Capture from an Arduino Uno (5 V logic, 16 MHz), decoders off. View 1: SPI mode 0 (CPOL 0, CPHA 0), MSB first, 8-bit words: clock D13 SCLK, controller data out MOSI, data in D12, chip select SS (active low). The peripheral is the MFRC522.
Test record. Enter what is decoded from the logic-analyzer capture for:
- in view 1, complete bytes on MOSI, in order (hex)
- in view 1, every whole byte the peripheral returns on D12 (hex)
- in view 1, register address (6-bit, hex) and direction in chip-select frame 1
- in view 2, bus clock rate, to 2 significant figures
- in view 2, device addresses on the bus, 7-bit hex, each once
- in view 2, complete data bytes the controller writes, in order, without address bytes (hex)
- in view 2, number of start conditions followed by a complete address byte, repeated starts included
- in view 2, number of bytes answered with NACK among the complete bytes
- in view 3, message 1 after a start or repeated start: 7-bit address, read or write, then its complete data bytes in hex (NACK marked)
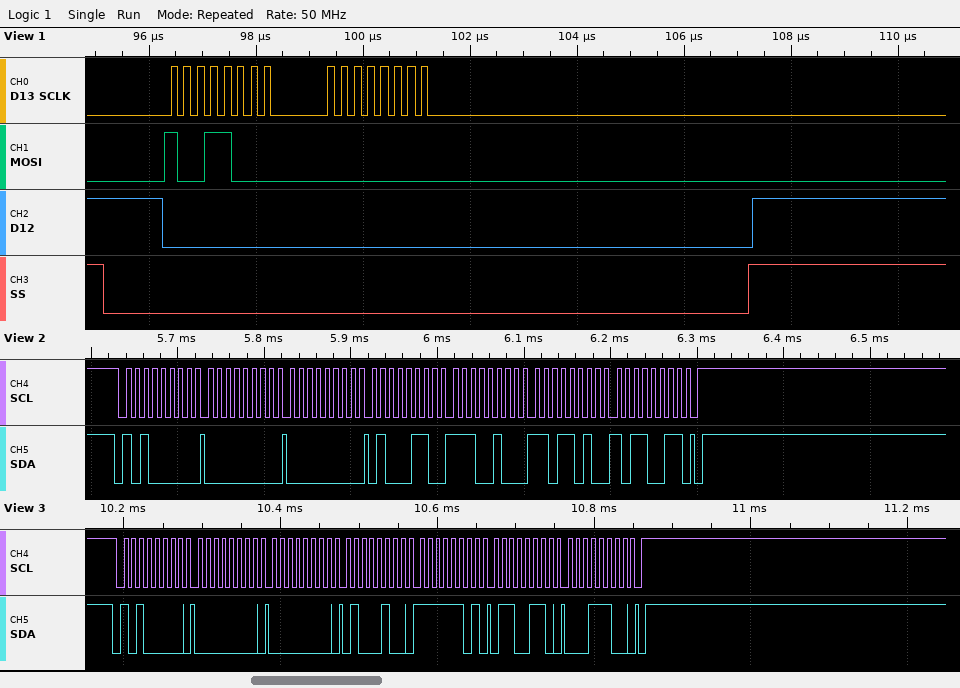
98 00
00 00
0x0C read
100 kHz
0x50
00 00 46 E4 DA B3
1
0
0x50 write: 00 00 44 FD 66 1C
